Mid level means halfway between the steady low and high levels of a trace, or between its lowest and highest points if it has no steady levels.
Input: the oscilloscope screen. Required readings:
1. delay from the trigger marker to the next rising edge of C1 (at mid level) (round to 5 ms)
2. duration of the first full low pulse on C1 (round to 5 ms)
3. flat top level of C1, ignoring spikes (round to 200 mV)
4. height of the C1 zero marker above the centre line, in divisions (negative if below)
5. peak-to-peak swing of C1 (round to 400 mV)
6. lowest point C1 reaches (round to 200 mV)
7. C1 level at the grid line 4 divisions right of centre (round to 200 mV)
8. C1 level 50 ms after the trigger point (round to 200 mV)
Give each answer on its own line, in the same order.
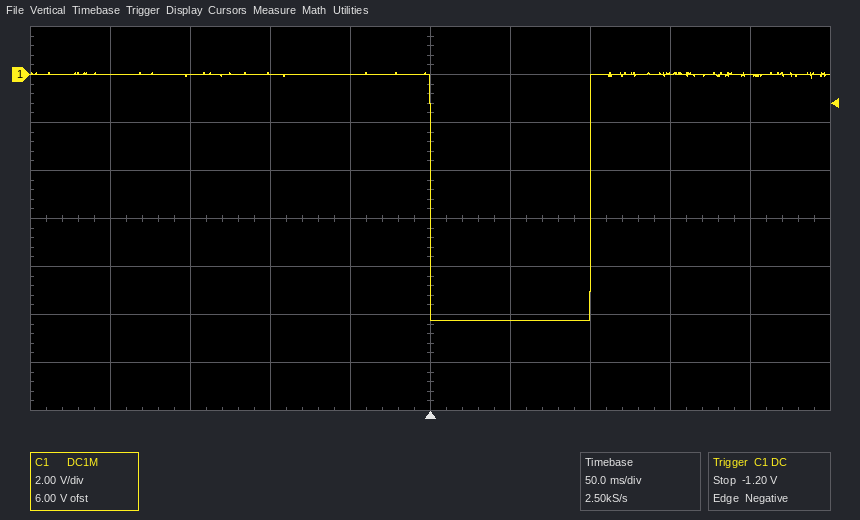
100 ms
100 ms
0.0 V
+3.0 div
10.4 V
-10.2 V
0.0 V
-10.2 V
